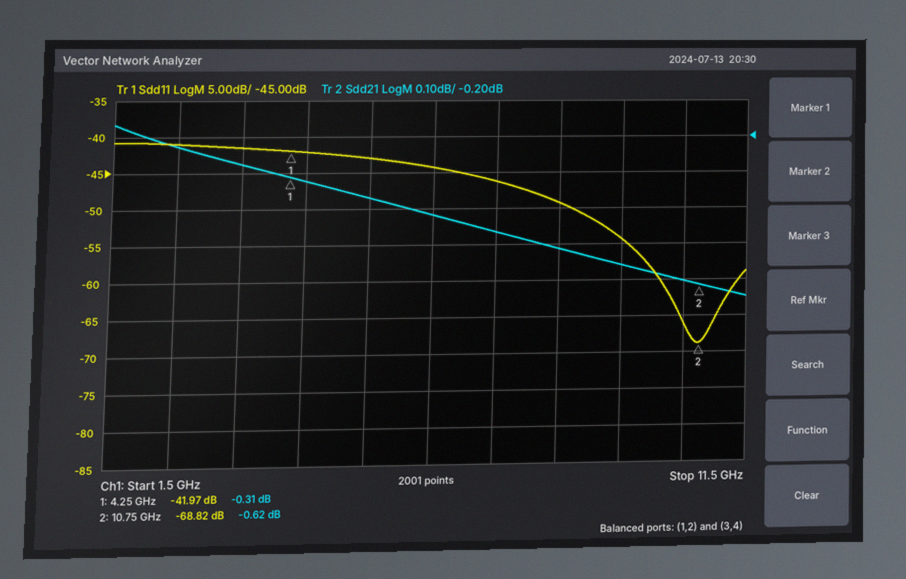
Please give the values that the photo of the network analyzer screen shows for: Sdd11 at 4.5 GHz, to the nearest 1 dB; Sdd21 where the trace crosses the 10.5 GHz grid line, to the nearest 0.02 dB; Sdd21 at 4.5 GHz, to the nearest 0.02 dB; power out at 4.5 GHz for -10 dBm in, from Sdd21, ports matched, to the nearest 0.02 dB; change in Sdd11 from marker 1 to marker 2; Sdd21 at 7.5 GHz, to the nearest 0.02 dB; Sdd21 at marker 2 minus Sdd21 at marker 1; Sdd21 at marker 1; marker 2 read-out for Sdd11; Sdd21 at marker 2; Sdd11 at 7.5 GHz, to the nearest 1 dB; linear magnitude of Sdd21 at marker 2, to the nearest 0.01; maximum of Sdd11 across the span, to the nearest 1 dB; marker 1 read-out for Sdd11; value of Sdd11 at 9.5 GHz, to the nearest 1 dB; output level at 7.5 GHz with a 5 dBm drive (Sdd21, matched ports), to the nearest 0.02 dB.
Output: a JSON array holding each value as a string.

["-42 dB", "-0.60 dB", "-0.32 dB", "-10.32 dBm", "-26.85 dB", "-0.46 dB", "-0.31 dB", "-0.31 dB", "-68.82 dB", "-0.62 dB", "-46 dB", "0.93", "-41 dB", "-41.97 dB", "-54 dB", "4.54 dBm"]
